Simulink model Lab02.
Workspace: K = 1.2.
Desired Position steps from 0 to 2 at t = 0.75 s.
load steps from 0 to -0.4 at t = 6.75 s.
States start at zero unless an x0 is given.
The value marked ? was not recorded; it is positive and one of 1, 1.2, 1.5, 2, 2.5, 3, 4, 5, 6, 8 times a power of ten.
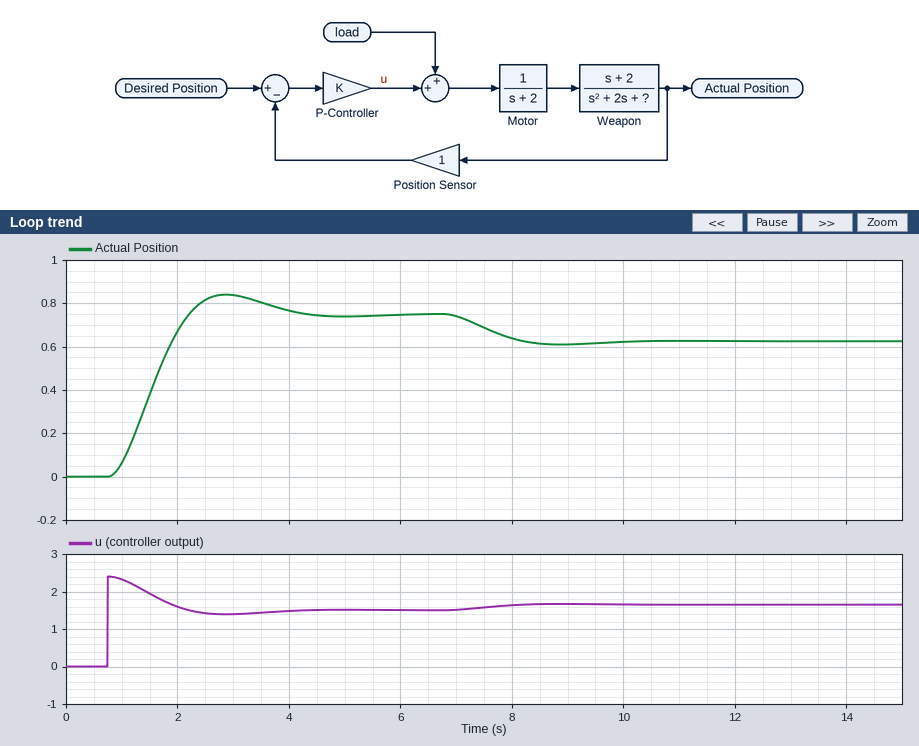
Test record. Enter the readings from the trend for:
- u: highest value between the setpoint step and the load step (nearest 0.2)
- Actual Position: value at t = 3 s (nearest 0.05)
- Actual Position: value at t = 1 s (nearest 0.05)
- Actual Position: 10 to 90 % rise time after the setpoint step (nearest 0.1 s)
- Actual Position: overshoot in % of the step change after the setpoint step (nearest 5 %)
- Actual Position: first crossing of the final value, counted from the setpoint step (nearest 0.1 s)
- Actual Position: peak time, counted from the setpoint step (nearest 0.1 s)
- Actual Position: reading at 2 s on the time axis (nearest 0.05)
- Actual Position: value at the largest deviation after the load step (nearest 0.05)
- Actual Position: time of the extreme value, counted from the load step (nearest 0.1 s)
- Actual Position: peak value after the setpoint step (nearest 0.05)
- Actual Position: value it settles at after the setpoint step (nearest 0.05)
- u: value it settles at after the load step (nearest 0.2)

2.4
0.85
0.05
1.0 s
10 %
1.5 s
2.1 s
0.65
0.60
2.1 s
0.85
0.75
1.6
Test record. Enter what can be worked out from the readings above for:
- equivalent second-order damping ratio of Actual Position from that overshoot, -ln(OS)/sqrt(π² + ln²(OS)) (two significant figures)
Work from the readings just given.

0.59
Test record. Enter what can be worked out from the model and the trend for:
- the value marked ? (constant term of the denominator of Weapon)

2
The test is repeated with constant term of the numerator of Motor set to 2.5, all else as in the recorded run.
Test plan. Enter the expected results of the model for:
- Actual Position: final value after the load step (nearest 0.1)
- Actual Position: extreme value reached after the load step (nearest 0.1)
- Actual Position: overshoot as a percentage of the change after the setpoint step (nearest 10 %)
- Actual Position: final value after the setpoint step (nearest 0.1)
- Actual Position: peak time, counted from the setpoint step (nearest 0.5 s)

1.0
1.0
20 %
1.2
1.5 s
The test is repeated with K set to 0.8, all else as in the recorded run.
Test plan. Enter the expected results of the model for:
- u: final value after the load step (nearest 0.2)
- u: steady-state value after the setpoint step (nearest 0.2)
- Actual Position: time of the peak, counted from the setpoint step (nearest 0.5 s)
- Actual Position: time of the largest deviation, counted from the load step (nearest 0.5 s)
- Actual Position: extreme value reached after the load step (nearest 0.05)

1.2
1.2
2.5 s
2.5 s
0.40
